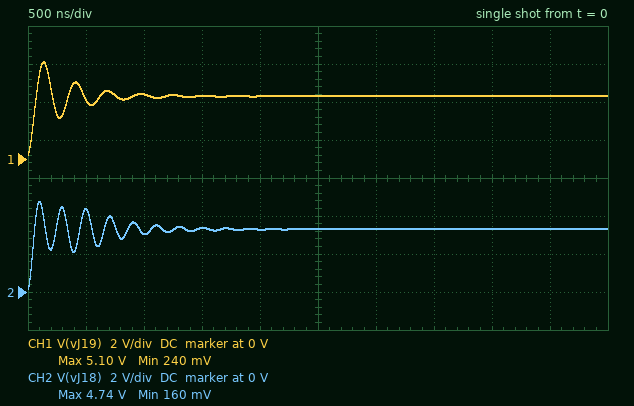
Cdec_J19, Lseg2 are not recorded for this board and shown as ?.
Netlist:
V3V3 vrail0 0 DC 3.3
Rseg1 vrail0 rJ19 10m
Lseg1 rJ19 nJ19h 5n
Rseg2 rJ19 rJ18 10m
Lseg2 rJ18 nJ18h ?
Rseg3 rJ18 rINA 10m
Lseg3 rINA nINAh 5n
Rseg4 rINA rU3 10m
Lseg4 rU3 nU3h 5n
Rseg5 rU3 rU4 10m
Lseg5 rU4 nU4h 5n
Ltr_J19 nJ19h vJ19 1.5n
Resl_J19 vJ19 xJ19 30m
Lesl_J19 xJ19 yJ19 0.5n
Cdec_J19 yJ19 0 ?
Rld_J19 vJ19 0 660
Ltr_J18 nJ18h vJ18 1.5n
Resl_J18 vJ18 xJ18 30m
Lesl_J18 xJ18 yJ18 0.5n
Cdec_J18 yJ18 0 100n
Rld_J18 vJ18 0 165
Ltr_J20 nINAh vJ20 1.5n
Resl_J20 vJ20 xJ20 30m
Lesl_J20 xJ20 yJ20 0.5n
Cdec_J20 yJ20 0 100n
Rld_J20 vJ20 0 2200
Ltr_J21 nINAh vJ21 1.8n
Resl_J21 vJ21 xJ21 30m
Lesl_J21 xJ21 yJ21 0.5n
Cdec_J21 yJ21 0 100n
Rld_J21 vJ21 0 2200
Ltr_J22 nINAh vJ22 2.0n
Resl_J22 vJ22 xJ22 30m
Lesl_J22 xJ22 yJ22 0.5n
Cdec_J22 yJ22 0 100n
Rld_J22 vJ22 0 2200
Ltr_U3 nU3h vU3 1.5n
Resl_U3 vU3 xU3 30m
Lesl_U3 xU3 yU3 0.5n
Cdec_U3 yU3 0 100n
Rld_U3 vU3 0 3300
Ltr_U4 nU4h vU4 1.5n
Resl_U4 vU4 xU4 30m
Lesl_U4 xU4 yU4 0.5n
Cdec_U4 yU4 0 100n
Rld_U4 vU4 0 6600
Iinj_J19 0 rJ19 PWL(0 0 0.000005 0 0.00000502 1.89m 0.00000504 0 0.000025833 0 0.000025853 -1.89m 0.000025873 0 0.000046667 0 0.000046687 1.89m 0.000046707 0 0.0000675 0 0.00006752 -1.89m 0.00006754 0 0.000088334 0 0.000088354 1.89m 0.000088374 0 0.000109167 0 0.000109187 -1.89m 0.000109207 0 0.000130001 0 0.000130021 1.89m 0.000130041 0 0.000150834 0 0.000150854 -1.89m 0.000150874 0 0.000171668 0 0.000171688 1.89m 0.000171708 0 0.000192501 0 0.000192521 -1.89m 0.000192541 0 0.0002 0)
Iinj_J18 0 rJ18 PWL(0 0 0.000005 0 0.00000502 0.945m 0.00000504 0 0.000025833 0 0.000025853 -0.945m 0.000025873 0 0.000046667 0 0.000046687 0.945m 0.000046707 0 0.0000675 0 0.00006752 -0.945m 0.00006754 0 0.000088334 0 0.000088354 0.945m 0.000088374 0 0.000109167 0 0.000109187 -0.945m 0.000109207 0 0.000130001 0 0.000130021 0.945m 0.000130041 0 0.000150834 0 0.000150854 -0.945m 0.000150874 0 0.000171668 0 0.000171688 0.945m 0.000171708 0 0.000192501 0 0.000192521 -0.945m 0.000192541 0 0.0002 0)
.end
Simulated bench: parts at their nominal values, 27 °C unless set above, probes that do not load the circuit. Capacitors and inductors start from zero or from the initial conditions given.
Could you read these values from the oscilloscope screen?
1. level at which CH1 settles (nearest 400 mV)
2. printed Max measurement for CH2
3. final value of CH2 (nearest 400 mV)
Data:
3.2 V
4.74 V
3.2 V
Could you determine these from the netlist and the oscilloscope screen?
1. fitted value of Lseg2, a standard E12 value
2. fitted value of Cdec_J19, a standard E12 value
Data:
8.2 nH
270 nF
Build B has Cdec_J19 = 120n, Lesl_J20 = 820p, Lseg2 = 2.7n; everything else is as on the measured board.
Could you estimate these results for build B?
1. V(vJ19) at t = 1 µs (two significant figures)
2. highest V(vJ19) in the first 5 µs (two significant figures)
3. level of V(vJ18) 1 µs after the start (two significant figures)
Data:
3.5 V
5.2 V
3.3 V
